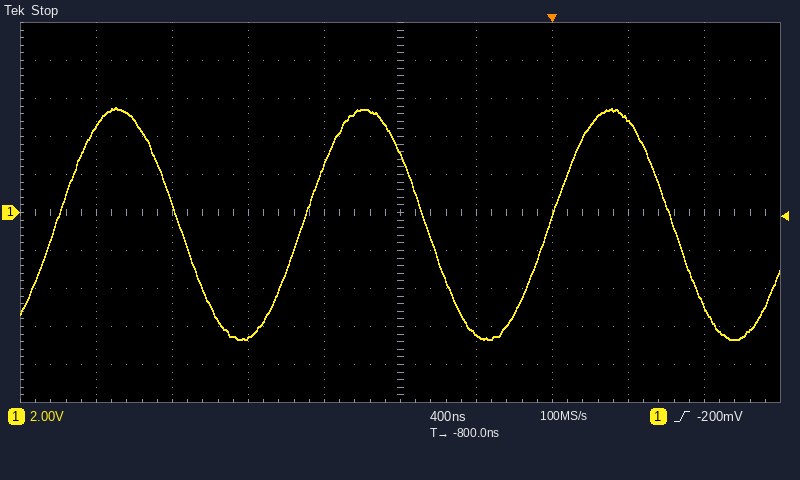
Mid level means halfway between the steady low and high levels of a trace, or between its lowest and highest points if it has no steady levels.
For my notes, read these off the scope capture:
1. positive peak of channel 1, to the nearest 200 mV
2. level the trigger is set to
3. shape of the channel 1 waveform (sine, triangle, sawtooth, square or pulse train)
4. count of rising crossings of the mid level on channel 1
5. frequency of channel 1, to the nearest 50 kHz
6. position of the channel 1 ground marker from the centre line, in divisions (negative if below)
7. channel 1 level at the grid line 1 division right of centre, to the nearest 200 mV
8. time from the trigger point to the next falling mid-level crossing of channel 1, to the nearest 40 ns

5.6 V
-200 mV
sine
3
750 kHz
0.0 div
-6.4 V
640 ns
